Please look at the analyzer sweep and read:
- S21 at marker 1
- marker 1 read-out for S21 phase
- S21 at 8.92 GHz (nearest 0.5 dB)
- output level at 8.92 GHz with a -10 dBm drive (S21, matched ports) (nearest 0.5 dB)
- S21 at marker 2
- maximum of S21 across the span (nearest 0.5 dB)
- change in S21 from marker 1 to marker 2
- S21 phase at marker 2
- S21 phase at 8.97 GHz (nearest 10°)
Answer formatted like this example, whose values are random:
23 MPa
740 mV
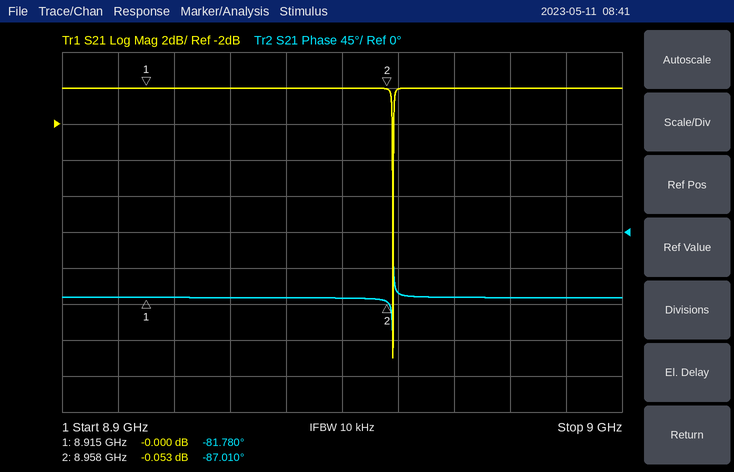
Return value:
-0.000 dB
-81.780°
0.0 dB
-10.0 dBm
-0.053 dB
0.0 dB
-0.053 dB
-87.010°
-80°
